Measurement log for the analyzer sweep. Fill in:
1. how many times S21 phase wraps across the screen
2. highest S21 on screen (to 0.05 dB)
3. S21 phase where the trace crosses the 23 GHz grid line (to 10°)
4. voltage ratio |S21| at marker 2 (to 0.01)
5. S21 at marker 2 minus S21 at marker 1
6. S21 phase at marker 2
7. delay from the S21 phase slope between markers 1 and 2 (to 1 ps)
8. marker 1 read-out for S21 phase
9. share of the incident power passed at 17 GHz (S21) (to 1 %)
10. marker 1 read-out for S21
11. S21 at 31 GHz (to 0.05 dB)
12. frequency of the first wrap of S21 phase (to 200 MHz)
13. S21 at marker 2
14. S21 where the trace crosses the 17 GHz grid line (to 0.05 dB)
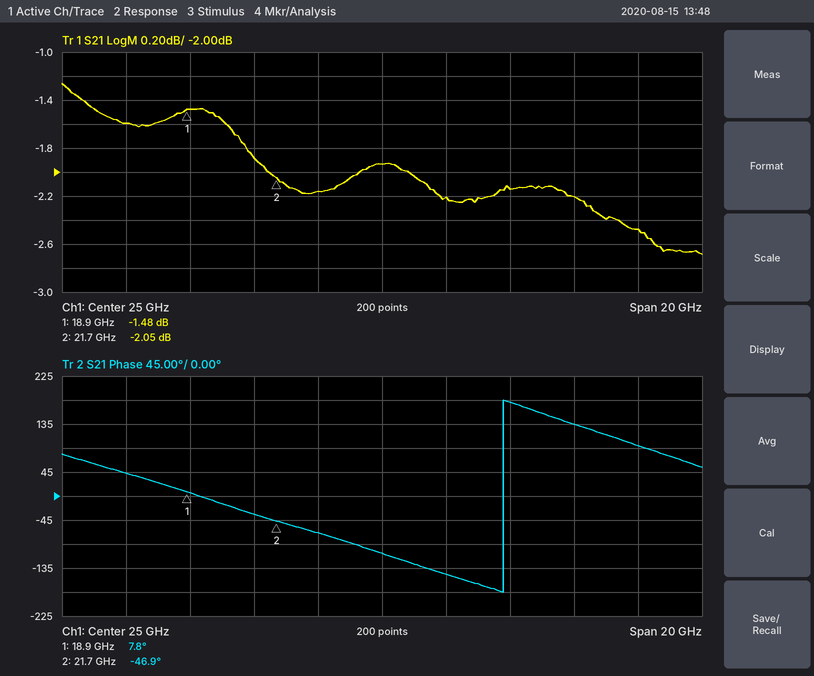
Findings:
1
-1.25 dB
-70°
0.79
-0.57 dB
-46.9°
54 ps
7.8°
69 %
-1.48 dB
-2.20 dB
28.8 GHz
-2.05 dB
-1.60 dB
